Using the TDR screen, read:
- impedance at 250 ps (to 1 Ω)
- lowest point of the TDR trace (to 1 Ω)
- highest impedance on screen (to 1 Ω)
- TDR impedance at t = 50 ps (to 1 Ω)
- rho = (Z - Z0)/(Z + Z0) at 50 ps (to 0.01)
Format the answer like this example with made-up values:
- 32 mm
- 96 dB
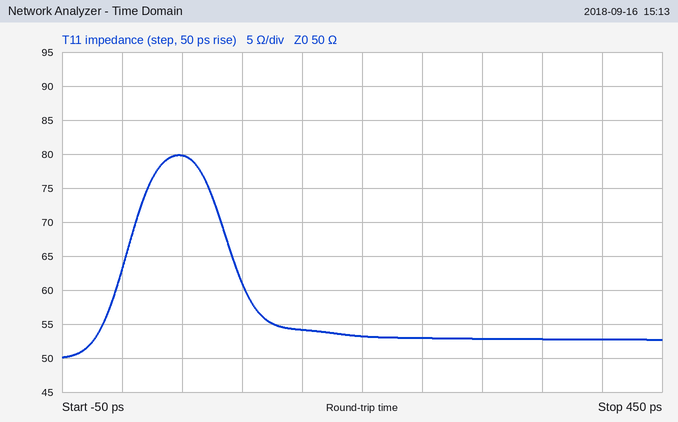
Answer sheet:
- 53 Ω
- 50 Ω
- 80 Ω
- 80 Ω
- +0.23
